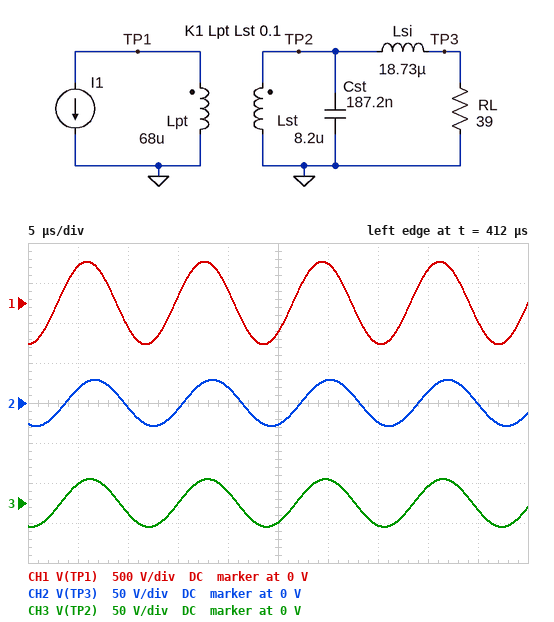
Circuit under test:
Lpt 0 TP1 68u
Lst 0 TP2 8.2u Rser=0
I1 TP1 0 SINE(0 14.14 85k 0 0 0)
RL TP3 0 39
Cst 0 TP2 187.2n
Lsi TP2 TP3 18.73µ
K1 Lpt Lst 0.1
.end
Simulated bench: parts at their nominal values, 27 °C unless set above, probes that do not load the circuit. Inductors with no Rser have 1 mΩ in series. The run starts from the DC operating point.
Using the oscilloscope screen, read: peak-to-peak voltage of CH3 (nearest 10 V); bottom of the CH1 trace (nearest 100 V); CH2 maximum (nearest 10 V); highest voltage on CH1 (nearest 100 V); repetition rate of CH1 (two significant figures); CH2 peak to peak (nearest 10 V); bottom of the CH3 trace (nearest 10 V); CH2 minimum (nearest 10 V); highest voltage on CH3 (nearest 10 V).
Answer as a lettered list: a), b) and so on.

a) 60 V
b) -500 V
c) 30 V
d) 500 V
e) 85 kHz
f) 60 V
g) -30 V
h) -30 V
i) 30 V
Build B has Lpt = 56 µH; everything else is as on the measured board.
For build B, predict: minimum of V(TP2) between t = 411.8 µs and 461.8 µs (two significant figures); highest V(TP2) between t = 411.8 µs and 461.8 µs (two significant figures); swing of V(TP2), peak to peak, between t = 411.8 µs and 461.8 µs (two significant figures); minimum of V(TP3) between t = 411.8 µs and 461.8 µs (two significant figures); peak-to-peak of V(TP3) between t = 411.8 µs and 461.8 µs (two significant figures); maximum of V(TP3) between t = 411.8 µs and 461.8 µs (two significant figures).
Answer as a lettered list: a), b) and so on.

a) -27 V
b) 27 V
c) 54 V
d) -26 V
e) 52 V
f) 26 V
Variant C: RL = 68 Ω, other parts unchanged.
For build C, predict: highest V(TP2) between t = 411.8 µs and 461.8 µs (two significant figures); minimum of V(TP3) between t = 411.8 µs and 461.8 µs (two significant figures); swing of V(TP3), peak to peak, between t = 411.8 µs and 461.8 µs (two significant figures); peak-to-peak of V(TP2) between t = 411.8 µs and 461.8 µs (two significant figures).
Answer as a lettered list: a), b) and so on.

a) 31 V
b) -31 V
c) 61 V
d) 62 V
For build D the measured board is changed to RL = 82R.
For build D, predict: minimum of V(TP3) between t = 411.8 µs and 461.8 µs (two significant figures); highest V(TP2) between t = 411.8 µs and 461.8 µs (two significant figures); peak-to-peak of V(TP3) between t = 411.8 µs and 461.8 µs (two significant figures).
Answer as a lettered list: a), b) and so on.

a) -31 V
b) 31 V
c) 62 V
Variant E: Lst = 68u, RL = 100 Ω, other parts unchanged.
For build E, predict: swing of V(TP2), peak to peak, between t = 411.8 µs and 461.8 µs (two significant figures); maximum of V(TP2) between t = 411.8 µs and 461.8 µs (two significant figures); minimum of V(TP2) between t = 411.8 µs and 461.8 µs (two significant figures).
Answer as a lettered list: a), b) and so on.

a) 39 V
b) 20 V
c) -20 V
